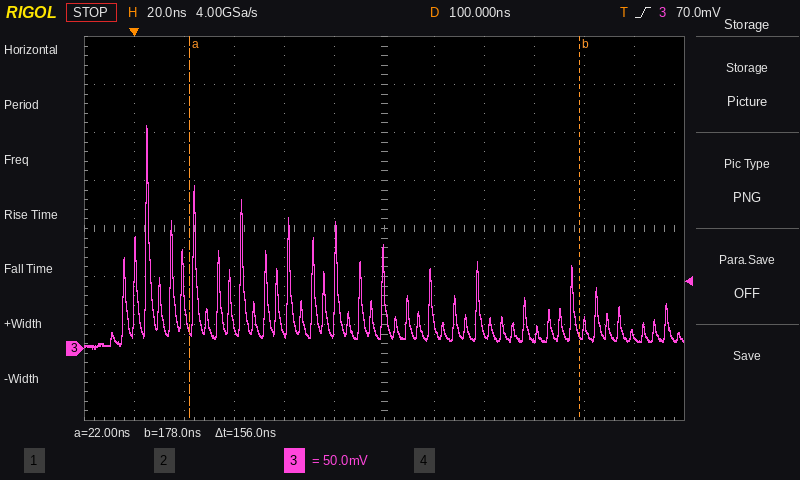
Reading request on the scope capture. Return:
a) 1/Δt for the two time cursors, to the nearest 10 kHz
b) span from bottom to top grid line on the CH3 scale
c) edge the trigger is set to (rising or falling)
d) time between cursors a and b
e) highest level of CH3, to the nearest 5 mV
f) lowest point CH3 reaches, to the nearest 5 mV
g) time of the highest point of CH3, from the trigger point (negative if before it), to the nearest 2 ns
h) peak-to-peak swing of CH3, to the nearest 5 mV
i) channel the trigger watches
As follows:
6.41 MHz
400 mV
rising
156 ns
230 mV
0 mV
+6 ns
230 mV
CH3
